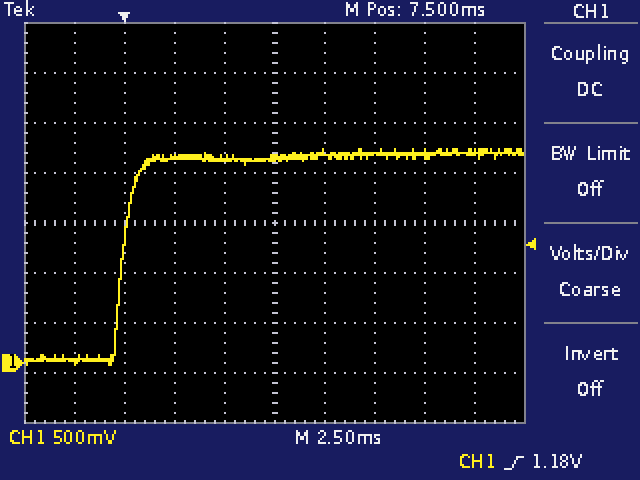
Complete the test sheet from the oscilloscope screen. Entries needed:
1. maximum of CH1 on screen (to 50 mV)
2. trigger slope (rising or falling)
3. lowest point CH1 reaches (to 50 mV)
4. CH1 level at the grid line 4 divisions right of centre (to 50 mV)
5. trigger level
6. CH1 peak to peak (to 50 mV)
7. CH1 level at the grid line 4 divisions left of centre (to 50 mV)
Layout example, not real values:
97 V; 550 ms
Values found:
2.15 V; rising; 0 mV; 2.10 V; 1.18 V; 2.15 V; 0 mV
